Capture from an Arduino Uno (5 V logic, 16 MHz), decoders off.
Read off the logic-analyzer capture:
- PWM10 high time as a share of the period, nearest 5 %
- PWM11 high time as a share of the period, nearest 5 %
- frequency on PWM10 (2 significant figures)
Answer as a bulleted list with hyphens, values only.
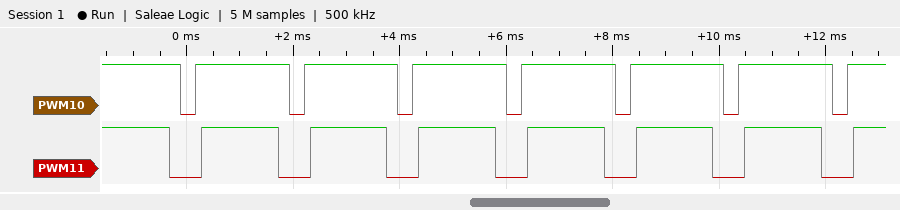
- 85 %
- 70 %
- 490 Hz
